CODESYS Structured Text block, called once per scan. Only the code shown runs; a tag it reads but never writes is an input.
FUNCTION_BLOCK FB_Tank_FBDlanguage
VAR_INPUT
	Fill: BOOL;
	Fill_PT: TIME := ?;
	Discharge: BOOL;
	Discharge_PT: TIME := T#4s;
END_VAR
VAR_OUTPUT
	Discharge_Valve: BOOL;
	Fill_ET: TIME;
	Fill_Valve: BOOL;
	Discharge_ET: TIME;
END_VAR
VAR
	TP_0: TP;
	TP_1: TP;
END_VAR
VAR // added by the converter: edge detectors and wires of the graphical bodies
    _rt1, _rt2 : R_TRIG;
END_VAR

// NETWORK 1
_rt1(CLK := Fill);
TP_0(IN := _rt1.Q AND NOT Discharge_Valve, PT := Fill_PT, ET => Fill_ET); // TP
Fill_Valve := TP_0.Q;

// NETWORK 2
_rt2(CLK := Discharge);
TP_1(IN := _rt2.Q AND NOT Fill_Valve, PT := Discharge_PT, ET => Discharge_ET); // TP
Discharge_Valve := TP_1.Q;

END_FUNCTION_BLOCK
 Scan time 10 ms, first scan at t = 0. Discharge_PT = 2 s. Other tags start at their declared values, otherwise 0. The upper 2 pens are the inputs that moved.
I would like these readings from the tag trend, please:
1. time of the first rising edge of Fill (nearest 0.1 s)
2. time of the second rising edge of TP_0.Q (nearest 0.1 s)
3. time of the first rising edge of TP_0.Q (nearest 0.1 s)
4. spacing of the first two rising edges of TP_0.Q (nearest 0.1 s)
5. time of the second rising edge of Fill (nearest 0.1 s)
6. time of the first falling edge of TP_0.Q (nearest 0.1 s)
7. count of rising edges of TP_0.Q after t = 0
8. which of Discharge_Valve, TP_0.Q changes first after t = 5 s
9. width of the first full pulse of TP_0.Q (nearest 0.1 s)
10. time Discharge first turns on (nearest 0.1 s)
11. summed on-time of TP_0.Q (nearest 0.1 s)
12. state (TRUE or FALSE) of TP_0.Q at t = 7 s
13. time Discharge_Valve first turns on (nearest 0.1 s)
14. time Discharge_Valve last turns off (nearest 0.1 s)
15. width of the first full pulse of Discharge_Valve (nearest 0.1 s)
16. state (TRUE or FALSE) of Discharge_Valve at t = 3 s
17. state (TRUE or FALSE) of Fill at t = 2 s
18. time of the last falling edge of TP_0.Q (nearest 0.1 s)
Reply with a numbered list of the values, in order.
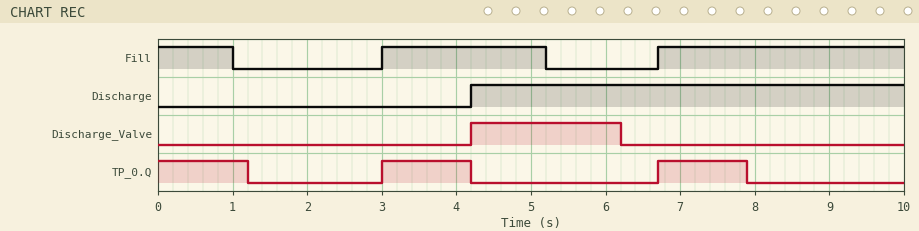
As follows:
1. 3.0 s
2. 6.7 s
3. 3.0 s
4. 3.7 s
5. 6.7 s
6. 1.2 s
7. 2
8. Discharge_Valve
9. 1.2 s
10. 4.2 s
11. 3.6 s
12. TRUE
13. 4.2 s
14. 6.2 s
15. 2.0 s
16. FALSE
17. FALSE
18. 7.9 s
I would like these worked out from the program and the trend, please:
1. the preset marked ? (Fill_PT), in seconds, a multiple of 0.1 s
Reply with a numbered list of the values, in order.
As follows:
1. 1.2 s
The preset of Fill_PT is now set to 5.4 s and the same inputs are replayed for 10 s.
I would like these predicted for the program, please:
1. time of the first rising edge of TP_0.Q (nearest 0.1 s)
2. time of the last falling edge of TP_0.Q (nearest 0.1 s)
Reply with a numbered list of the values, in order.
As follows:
1. 6.7 s
2. 5.4 s
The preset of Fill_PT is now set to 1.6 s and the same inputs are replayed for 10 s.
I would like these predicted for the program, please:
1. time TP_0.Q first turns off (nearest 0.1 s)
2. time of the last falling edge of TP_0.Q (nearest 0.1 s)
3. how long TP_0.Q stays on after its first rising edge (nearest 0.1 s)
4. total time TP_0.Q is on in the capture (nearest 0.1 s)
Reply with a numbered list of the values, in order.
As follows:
1. 1.6 s
2. 8.3 s
3. 1.6 s
4. 4.8 s
